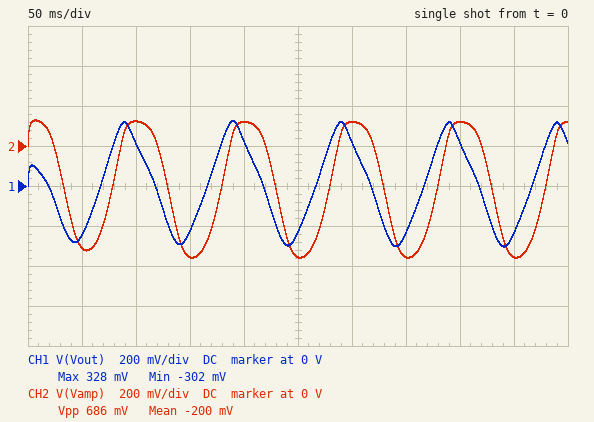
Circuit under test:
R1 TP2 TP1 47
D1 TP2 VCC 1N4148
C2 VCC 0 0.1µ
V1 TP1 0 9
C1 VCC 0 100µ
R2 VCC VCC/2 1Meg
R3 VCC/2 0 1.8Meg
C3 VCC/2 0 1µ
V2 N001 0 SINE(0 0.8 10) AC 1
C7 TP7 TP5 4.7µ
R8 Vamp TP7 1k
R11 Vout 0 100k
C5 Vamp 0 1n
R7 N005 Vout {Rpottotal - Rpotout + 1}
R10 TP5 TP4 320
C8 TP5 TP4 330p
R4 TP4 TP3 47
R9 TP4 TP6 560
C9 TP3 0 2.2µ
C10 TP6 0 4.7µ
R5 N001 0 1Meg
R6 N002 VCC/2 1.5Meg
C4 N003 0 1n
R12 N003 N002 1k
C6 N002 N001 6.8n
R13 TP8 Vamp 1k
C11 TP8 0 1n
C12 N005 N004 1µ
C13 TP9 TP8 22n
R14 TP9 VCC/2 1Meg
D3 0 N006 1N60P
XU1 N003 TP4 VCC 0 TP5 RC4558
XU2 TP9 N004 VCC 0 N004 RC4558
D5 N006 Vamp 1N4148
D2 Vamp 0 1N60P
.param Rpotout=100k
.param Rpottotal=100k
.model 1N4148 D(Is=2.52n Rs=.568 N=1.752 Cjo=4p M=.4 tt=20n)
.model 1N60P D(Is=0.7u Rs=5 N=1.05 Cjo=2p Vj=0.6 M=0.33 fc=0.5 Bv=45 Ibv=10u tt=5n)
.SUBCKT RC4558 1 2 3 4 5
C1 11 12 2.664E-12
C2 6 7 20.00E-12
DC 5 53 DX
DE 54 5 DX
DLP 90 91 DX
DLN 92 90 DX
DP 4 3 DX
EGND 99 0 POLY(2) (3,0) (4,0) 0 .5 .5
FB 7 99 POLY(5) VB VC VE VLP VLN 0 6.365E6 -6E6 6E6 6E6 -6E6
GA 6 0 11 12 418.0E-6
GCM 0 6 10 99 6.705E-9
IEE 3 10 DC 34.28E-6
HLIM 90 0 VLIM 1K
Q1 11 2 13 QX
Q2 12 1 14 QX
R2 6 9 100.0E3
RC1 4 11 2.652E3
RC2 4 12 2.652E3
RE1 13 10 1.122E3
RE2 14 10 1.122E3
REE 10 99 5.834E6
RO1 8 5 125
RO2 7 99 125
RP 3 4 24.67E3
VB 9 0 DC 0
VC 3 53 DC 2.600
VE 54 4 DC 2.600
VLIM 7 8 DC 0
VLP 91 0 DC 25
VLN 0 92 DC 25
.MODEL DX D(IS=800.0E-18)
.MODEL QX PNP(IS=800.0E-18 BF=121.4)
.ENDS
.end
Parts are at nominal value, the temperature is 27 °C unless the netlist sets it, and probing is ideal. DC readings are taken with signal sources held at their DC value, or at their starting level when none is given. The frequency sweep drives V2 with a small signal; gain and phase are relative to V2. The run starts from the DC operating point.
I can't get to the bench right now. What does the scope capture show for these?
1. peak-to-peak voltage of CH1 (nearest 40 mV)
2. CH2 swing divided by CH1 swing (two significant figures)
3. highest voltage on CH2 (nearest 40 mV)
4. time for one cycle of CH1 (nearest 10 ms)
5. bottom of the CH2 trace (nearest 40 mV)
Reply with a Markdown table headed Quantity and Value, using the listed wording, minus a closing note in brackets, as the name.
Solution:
| Quantity | Value |
|---|---|
| peak-to-peak voltage of CH1 | 640 mV |
| CH2 swing divided by CH1 swing | 1.1 |
| highest voltage on CH2 | 120 mV |
| time for one cycle of CH1 | 100 ms |
| bottom of the CH2 trace | -560 mV |
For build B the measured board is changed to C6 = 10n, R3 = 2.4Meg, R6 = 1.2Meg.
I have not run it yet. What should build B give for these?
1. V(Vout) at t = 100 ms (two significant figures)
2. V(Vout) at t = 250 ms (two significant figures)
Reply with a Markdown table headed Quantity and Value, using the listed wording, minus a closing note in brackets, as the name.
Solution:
| Quantity | Value |
|---|---|
| V(Vout) at t = 100 ms | 130 mV |
| V(Vout) at t = 250 ms | -260 mV |
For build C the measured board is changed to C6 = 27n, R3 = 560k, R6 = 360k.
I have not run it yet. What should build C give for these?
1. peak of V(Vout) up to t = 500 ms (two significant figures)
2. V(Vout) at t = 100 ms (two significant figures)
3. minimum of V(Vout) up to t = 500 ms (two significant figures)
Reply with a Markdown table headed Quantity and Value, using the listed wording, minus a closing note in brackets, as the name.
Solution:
| Quantity | Value |
|---|---|
| peak of V(Vout) up to t = 500 ms | 320 mV |
| V(Vout) at t = 100 ms | 200 mV |
| minimum of V(Vout) up to t = 500 ms | -290 mV |
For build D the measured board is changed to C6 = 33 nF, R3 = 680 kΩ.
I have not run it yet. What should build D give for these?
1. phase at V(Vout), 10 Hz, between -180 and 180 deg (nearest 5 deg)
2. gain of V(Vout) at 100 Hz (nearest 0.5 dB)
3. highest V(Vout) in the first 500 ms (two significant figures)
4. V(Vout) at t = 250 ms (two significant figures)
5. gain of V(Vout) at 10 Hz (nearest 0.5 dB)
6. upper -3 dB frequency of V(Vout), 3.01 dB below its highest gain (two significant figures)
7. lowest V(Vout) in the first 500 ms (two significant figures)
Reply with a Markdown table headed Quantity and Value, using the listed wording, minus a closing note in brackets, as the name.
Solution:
| Quantity | Value |
|---|---|
| phase at V(Vout), 10 Hz, between -180 and 180 deg | 75 deg |
| gain of V(Vout) at 100 Hz | 3.5 dB |
| highest V(Vout) in the first 500 ms | 450 mV |
| V(Vout) at t = 250 ms | -350 mV |
| gain of V(Vout) at 10 Hz | -3.0 dB |
| upper -3 dB frequency of V(Vout), 3.01 dB below its highest gain | 55 kHz |
| lowest V(Vout) in the first 500 ms | -420 mV |
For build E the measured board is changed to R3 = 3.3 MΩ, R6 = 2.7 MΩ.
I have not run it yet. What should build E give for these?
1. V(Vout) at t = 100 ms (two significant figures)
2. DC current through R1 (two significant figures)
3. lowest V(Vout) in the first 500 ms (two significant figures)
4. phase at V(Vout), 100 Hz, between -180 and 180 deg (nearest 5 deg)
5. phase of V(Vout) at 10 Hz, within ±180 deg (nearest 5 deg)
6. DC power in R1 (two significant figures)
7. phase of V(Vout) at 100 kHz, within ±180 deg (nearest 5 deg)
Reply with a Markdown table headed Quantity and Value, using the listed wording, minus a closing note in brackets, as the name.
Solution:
| Quantity | Value |
|---|---|
| V(Vout) at t = 100 ms | 10 mV |
| DC current through R1 | 690 µA |
| lowest V(Vout) in the first 500 ms | -56 mV |
| phase at V(Vout), 100 Hz, between -180 and 180 deg | 10 deg |
| phase of V(Vout) at 10 Hz, within ±180 deg | 80 deg |
| DC power in R1 | 22 µW |
| phase of V(Vout) at 100 kHz, within ±180 deg | 160 deg |
